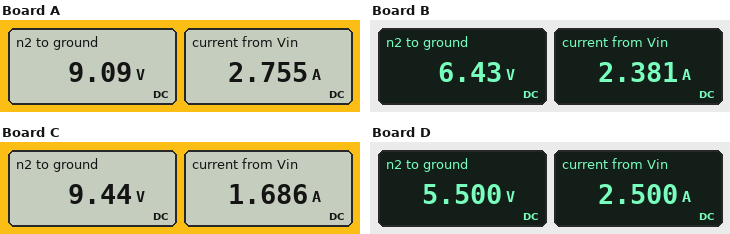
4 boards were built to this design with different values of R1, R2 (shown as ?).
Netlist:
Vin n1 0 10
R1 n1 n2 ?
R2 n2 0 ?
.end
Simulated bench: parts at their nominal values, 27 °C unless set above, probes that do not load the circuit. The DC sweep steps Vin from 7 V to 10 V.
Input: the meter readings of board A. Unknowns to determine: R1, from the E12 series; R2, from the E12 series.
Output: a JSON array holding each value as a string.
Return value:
["0.33 Ω", "3.3 Ω"]
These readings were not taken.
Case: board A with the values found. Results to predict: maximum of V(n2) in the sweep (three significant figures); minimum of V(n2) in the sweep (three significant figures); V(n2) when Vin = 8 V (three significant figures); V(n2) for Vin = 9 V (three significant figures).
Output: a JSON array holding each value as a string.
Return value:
["9.09 V", "6.36 V", "7.27 V", "8.18 V"]
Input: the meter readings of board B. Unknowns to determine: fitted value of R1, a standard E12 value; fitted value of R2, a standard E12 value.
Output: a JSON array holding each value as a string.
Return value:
["1.5 Ω", "2.7 Ω"]
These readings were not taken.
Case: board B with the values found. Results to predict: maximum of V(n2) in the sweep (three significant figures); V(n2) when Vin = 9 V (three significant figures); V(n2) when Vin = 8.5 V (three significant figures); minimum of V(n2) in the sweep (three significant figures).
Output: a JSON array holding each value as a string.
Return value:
["6.43 V", "5.79 V", "5.46 V", "4.50 V"]
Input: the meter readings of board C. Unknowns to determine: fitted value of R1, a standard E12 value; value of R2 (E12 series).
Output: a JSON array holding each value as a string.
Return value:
["0.33 Ω", "5.6 Ω"]
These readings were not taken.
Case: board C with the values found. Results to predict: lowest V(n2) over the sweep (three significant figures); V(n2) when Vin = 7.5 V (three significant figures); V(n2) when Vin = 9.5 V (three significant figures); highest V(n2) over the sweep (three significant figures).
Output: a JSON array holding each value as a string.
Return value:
["6.61 V", "7.08 V", "8.97 V", "9.44 V"]
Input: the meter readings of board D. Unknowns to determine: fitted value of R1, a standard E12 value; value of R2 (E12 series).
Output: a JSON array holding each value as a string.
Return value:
["1.8 Ω", "2.2 Ω"]
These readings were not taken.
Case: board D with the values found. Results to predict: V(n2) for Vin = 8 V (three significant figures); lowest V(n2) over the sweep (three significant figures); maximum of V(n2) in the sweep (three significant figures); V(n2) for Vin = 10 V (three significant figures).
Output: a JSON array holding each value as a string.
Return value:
["4.40 V", "3.85 V", "5.50 V", "5.50 V"]
